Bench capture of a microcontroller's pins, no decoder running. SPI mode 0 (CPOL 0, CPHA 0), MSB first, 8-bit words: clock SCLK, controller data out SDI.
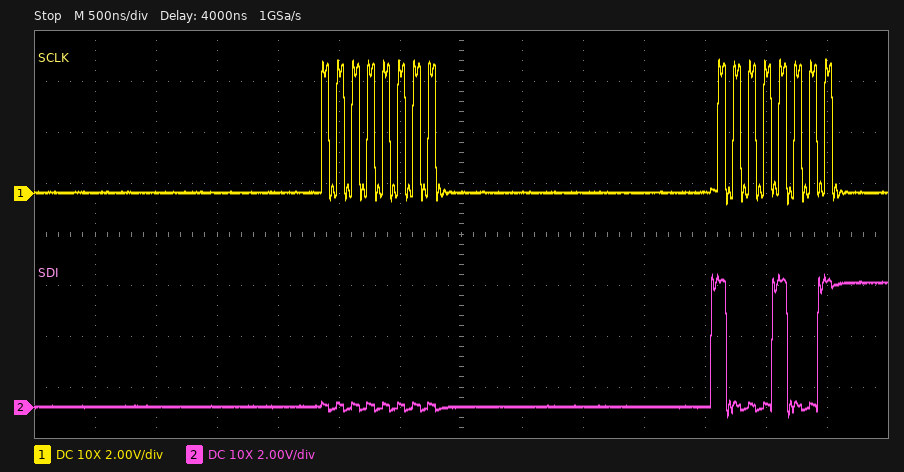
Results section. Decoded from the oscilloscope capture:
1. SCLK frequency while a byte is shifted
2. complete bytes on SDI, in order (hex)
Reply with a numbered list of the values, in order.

1. 8 MHz
2. 00 89
